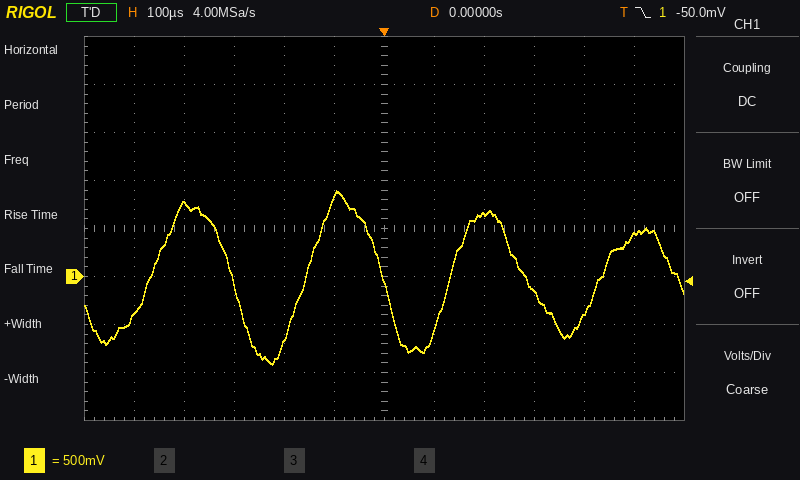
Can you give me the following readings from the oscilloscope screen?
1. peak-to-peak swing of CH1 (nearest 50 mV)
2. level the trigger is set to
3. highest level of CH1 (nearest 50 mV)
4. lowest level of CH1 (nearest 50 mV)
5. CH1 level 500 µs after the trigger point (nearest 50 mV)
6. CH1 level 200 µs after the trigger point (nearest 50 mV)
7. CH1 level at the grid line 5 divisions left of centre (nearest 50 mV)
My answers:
1.80 V
-50.0 mV
900 mV
-900 mV
450 mV
650 mV
-400 mV
